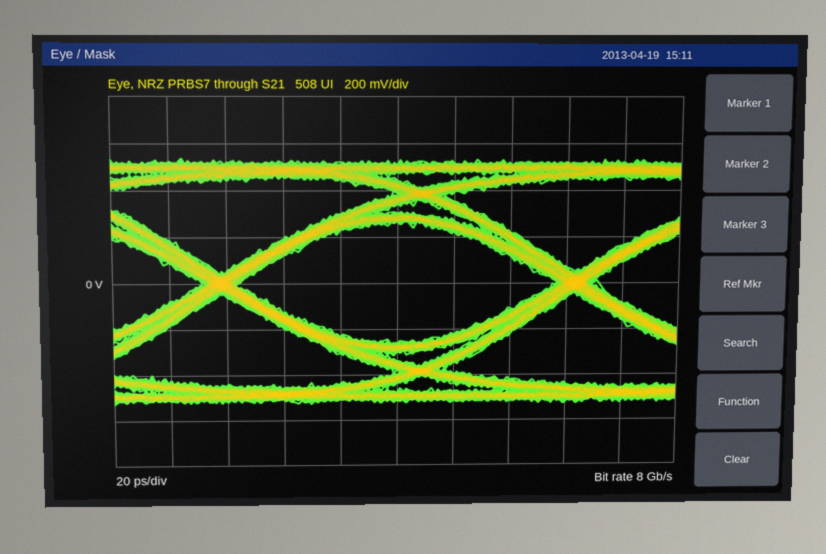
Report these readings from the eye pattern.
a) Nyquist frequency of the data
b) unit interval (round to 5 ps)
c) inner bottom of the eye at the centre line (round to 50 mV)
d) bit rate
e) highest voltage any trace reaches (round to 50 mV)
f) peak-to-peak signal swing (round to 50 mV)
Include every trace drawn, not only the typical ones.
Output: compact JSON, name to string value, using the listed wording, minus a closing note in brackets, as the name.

{"Nyquist frequency of the data": "4 GHz", "unit interval": "125 ps", "inner bottom of the eye at the centre line": "-250 mV", "bit rate": "8 Gb/s", "highest voltage any trace reaches": "550 mV", "peak-to-peak signal swing": "1.05 V"}
